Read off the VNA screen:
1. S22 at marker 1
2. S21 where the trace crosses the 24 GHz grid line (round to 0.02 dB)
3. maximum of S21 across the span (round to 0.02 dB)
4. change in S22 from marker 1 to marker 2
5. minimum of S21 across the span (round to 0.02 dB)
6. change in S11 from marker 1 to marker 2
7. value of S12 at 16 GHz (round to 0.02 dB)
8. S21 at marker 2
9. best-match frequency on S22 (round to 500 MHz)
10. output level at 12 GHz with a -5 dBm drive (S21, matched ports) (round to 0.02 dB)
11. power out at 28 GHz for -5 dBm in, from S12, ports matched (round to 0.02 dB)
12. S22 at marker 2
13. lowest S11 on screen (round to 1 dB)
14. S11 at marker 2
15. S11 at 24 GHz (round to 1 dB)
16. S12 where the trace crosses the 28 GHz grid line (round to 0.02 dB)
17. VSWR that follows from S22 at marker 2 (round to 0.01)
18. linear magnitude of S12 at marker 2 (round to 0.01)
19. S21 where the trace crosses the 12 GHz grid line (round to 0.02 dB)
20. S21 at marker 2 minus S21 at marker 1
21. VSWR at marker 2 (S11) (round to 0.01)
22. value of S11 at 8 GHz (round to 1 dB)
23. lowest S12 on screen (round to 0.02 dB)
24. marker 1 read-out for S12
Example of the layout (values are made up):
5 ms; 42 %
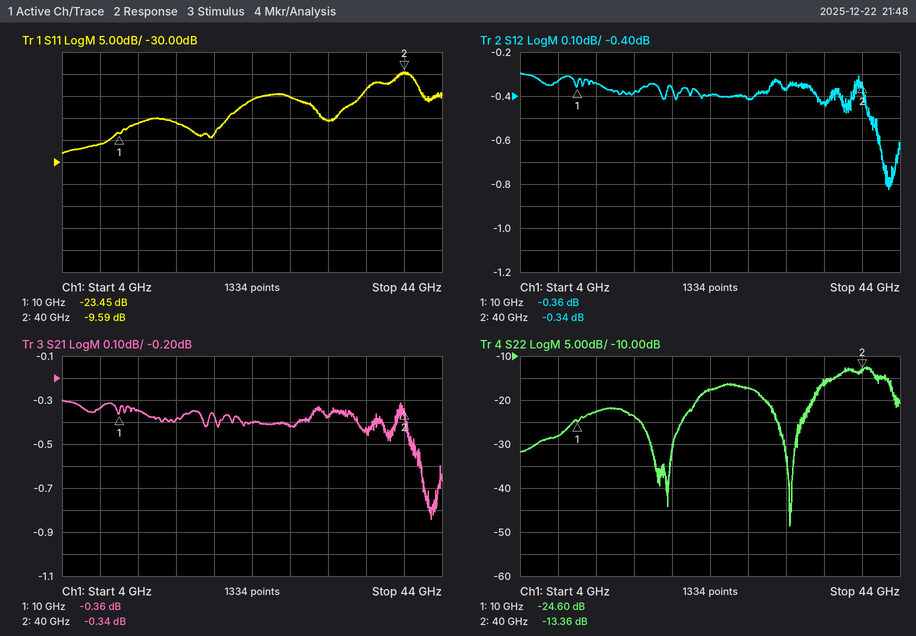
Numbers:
-24.60 dB; -0.40 dB; -0.30 dB; 11.24 dB; -0.84 dB; 13.86 dB; -0.38 dB; -0.34 dB; 32.5 GHz; -5.34 dBm; -5.42 dBm; -13.36 dB; -28 dB; -9.59 dB; -16 dB; -0.42 dB; 1.55; 0.96; -0.34 dB; 0.02 dB; 1.99; -26 dB; -0.82 dB; -0.36 dB
